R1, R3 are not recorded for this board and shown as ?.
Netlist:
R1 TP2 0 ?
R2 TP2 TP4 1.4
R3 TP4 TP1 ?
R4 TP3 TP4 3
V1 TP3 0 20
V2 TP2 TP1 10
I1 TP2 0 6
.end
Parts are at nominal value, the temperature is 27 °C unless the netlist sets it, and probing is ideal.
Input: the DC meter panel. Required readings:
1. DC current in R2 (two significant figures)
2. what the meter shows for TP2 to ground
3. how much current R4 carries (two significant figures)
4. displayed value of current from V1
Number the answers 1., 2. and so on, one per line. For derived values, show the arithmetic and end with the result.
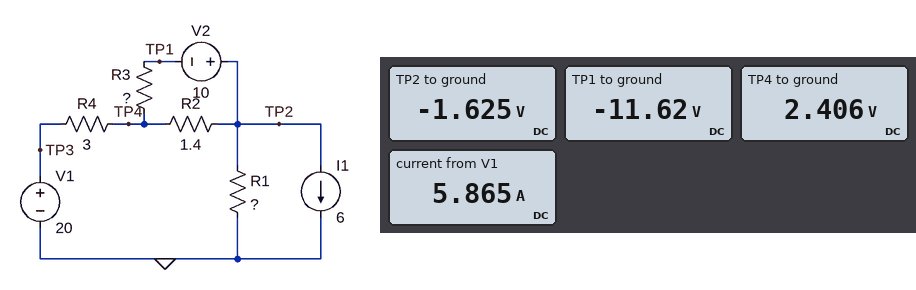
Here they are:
1. (2.406 V - (-1.625 V)) / 1.4 Ω = 2.9 A
2. -1.625 V
3. (20 V - 2.406 V) / 3 Ω = 5.9 A
4. 5.865 A
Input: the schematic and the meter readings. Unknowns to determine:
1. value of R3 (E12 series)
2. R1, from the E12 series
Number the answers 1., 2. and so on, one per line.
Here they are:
1. 4.7 Ω
2. 12 Ω
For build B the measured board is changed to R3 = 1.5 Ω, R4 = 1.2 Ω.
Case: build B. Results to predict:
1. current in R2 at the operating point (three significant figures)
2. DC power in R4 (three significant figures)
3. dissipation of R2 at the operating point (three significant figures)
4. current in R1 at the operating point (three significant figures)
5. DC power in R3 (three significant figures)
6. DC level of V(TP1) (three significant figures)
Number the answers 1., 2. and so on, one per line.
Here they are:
1. 149 mA
2. 58.0 W
3. 30.9 mW
4. 954 mA
5. 69.5 W
6. 1.45 V
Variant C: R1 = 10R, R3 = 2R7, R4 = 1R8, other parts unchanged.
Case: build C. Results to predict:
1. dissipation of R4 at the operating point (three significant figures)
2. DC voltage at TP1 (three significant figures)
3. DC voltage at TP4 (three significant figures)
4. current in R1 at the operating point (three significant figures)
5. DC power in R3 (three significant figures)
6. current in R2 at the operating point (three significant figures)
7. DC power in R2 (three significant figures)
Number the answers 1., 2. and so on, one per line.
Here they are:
1. 77.4 W
2. -4.43 V
3. 8.20 V
4. 557 mA
5. 59.1 W
6. 1.88 A
7. 4.94 W
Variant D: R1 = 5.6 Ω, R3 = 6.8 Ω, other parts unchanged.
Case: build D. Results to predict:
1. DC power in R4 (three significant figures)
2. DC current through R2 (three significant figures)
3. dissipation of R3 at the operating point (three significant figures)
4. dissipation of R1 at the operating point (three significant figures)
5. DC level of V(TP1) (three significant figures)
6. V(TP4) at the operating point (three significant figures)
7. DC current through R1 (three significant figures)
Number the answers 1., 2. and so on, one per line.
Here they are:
1. 96.3 W
2. 3.48 A
3. 32.5 W
4. 624 mW
5. -11.9 V
6. 3.00 V
7. 334 mA
